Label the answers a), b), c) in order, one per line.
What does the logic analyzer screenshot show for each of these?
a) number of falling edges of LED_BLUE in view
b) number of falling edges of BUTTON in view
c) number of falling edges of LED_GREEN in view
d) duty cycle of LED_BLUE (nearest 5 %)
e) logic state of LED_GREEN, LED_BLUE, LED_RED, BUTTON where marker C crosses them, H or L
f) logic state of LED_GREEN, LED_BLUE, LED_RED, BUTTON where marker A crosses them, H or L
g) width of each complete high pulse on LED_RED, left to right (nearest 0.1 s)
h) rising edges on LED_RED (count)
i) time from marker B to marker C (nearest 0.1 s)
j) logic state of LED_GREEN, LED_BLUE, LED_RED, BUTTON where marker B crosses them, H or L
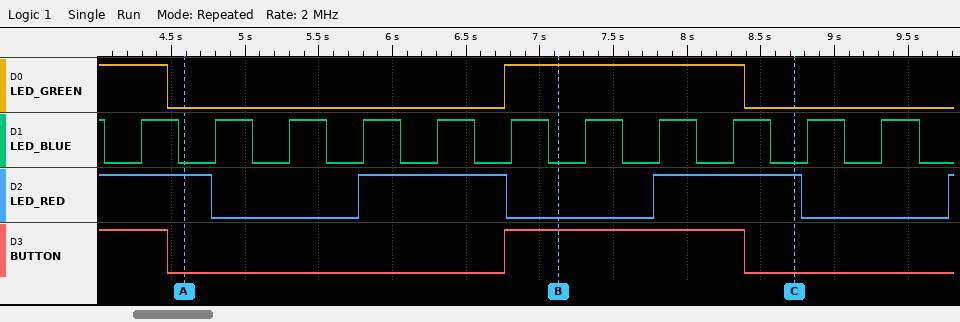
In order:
a) 12
b) 2
c) 2
d) 50 %
e) LED_GREEN=L, LED_BLUE=L, LED_RED=H, BUTTON=L
f) LED_GREEN=L, LED_BLUE=L, LED_RED=H, BUTTON=L
g) 1 s, 1 s
h) 3
i) 1.6 s
j) LED_GREEN=H, LED_BLUE=L, LED_RED=L, BUTTON=H
